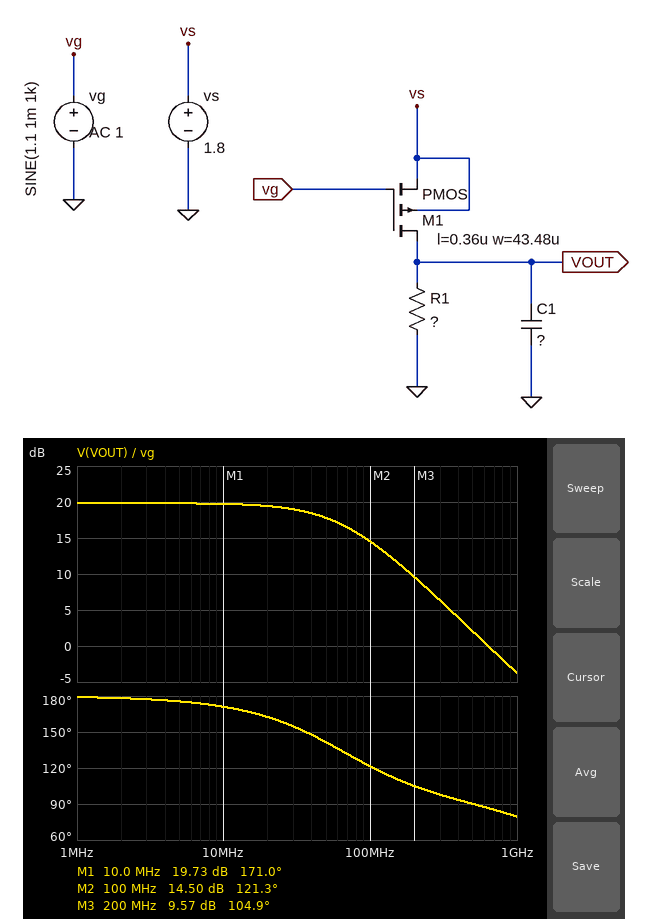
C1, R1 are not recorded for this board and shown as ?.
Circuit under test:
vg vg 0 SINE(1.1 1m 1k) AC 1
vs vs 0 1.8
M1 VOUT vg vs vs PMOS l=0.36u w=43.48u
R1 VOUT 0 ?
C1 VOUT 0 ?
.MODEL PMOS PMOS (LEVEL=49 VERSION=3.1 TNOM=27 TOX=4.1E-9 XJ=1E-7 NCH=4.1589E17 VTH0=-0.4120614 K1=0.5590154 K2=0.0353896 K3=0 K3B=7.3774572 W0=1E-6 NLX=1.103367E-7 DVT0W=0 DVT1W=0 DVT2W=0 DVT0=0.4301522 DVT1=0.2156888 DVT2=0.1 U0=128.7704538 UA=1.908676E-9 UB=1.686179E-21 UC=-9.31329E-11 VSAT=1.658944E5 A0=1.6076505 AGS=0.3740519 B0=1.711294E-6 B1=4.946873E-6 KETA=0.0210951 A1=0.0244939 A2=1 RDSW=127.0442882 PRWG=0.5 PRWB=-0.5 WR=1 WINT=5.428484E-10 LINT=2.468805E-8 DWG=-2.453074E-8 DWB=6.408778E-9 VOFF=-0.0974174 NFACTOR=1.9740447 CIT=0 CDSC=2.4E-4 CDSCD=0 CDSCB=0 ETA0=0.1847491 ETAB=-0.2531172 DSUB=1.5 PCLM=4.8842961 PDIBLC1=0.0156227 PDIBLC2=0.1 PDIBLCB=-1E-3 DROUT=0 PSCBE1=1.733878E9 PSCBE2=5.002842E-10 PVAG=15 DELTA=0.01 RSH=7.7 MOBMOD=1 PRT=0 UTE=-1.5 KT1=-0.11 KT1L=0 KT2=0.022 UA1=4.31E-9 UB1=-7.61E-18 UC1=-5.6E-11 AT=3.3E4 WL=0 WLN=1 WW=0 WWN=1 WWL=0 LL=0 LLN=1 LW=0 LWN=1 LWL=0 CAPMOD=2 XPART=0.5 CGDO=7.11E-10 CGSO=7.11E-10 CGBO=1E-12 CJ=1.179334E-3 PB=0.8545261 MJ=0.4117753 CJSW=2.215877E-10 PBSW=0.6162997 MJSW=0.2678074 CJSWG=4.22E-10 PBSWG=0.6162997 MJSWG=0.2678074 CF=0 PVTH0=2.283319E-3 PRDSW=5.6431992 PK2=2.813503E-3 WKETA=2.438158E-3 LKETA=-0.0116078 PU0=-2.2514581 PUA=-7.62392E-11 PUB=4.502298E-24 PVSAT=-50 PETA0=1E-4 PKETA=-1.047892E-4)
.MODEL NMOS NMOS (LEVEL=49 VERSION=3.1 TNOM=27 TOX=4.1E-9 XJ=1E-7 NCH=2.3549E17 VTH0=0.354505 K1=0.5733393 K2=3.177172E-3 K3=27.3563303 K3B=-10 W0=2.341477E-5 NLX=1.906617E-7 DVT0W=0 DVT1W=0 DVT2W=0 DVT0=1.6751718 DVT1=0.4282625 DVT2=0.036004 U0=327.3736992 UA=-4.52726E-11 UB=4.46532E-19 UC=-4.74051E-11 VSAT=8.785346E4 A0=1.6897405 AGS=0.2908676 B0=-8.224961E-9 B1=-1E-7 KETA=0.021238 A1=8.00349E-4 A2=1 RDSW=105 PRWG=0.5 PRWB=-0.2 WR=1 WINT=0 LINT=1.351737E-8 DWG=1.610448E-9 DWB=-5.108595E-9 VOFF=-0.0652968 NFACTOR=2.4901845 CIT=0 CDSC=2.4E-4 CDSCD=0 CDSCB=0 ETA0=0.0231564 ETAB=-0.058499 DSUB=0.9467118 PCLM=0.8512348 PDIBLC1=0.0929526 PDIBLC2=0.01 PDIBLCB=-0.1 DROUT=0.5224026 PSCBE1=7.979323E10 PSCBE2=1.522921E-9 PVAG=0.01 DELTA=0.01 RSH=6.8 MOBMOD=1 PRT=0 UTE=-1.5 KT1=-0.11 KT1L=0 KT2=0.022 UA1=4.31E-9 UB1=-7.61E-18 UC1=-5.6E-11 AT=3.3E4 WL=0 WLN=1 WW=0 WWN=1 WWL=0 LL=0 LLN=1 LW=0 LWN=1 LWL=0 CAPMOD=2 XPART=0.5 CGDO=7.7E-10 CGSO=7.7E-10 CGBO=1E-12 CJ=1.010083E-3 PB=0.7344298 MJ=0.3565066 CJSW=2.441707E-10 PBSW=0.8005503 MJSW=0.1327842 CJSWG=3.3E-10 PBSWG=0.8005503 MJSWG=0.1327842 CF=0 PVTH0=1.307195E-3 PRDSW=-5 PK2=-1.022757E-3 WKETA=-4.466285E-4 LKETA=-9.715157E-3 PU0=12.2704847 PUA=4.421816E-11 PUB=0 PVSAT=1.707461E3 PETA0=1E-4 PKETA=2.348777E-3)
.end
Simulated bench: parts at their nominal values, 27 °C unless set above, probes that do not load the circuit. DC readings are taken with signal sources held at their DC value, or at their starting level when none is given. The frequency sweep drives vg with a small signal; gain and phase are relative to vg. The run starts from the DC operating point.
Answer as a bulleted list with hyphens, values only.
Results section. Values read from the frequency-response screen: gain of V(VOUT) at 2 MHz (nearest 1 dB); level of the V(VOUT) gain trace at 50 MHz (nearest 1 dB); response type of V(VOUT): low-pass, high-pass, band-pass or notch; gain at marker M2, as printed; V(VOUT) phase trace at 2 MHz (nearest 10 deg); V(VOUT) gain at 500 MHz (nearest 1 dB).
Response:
- 20 dB
- 18 dB
- low-pass
- 14.50 dB
- 180 deg
- 2 dB
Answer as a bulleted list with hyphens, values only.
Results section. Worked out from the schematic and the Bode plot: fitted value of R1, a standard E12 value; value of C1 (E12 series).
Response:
- 6.8 kΩ
- 390 fF
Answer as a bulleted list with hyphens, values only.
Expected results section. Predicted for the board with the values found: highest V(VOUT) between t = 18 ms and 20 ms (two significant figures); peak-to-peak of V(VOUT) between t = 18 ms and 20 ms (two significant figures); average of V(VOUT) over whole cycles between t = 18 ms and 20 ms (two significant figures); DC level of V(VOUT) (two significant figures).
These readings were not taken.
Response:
- 1.5 V
- 20 mV
- 1.5 V
- 1.5 V
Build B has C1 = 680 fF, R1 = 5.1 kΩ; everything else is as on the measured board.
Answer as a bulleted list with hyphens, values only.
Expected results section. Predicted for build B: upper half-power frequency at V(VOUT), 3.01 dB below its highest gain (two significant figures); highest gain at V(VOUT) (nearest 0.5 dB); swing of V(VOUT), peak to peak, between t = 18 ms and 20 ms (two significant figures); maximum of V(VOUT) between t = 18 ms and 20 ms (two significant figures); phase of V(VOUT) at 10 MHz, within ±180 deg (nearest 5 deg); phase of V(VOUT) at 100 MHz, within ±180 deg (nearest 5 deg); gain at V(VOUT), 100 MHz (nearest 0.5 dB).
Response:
- 47 MHz
- 18.5 dB
- 17 mV
- 1.1 V
- 170 deg
- 115 deg
- 11.0 dB
